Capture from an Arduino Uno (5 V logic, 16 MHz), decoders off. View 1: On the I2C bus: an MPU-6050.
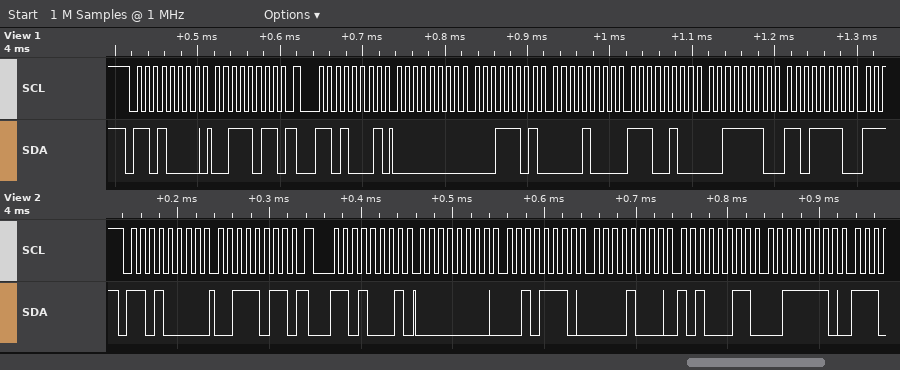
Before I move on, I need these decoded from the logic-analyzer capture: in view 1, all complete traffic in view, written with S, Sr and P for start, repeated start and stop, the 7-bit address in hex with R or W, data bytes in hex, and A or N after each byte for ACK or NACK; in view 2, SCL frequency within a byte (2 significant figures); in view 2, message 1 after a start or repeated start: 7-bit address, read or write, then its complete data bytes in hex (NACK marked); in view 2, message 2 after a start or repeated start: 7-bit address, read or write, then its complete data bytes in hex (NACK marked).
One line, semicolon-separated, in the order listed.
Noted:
S 68W A 3B A Sr 68R A 00 A 1D A 08 A E4 A 3E A DE A; 100 kHz; 0x68 write: 3B; 0x68 read: 00 2E 08 A3 3E
